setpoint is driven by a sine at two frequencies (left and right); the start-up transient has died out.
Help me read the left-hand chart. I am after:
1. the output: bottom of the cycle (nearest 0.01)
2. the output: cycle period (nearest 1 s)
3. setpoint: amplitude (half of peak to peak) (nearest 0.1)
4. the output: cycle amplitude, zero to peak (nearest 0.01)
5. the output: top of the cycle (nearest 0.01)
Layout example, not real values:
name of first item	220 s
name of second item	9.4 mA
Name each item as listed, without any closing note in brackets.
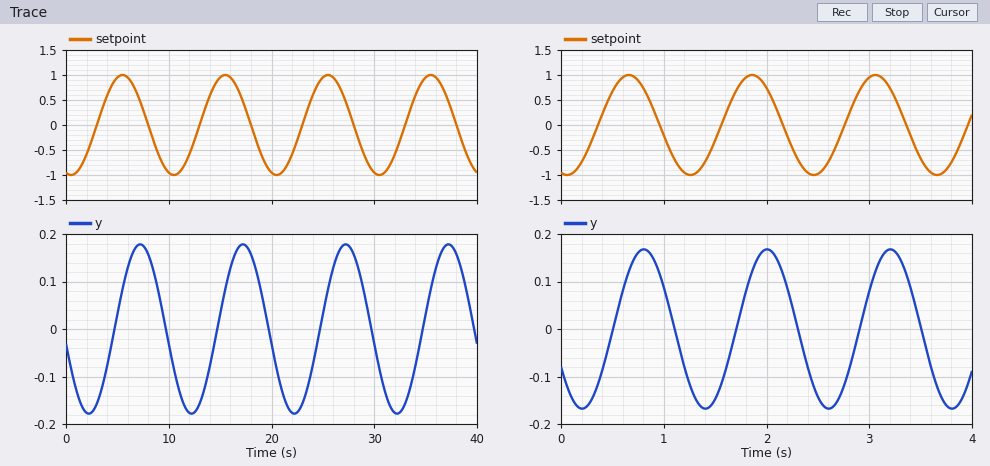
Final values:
the output: bottom of the cycle	-0.18
the output: cycle period	10 s
setpoint: amplitude (half of peak to peak)	1.0
the output: cycle amplitude, zero to peak	0.18
the output: top of the cycle	0.18
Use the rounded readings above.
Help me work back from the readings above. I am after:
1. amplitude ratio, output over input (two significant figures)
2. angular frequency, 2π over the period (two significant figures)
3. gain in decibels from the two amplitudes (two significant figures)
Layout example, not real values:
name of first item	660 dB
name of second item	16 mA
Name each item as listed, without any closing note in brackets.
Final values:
amplitude ratio, output over input	0.18
angular frequency, 2π over the period	0.63 rad/s
gain in decibels from the two amplitudes	-15 dB
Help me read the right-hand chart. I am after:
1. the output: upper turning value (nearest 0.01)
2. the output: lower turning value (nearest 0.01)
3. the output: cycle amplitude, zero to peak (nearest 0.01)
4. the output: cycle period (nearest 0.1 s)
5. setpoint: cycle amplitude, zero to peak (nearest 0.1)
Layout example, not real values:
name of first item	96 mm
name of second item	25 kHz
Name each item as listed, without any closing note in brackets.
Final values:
the output: upper turning value	0.17
the output: lower turning value	-0.17
the output: cycle amplitude, zero to peak	0.17
the output: cycle period	1.2 s
setpoint: cycle amplitude, zero to peak	1.0
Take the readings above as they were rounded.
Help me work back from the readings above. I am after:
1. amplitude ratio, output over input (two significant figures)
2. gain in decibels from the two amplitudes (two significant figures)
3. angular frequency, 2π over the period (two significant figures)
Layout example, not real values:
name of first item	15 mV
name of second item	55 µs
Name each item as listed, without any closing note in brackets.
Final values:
amplitude ratio, output over input	0.17
gain in decibels from the two amplitudes	-15 dB
angular frequency, 2π over the period	5.2 rad/s
